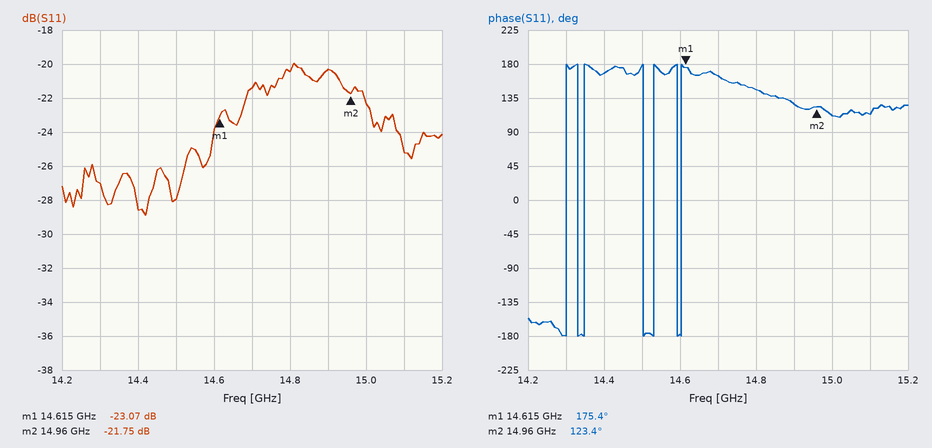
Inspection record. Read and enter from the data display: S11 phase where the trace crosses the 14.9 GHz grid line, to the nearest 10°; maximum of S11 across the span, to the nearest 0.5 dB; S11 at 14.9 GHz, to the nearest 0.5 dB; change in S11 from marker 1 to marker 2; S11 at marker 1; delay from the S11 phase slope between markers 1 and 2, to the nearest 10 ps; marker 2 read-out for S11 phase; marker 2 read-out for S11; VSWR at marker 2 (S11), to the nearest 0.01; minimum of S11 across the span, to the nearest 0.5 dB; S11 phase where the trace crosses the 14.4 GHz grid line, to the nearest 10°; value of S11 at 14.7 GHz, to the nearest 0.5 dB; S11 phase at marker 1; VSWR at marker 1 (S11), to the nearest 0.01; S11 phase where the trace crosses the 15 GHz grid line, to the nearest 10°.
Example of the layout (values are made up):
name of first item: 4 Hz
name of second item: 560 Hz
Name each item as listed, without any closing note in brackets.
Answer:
S11 phase where the trace crosses the 14.9 GHz grid line, to the nearest 10°: 130°
maximum of S11 across the span, to the nearest 0.5 dB: -20.0 dB
S11 at 14.9 GHz, to the nearest 0.5 dB: -20.5 dB
change in S11 from marker 1 to marker 2: 1.32 dB
S11 at marker 1: -23.07 dB
delay from the S11 phase slope between markers 1 and 2, to the nearest 10 ps: 420 ps
marker 2 read-out for S11 phase: 123.4°
marker 2 read-out for S11: -21.75 dB
VSWR at marker 2 (S11), to the nearest 0.01: 1.18
minimum of S11 across the span, to the nearest 0.5 dB: -29.0 dB
S11 phase where the trace crosses the 14.4 GHz grid line, to the nearest 10°: 170°
value of S11 at 14.7 GHz, to the nearest 0.5 dB: -21.5 dB
S11 phase at marker 1: 175.4°
VSWR at marker 1 (S11), to the nearest 0.01: 1.15
S11 phase where the trace crosses the 15 GHz grid line, to the nearest 10°: 110°
